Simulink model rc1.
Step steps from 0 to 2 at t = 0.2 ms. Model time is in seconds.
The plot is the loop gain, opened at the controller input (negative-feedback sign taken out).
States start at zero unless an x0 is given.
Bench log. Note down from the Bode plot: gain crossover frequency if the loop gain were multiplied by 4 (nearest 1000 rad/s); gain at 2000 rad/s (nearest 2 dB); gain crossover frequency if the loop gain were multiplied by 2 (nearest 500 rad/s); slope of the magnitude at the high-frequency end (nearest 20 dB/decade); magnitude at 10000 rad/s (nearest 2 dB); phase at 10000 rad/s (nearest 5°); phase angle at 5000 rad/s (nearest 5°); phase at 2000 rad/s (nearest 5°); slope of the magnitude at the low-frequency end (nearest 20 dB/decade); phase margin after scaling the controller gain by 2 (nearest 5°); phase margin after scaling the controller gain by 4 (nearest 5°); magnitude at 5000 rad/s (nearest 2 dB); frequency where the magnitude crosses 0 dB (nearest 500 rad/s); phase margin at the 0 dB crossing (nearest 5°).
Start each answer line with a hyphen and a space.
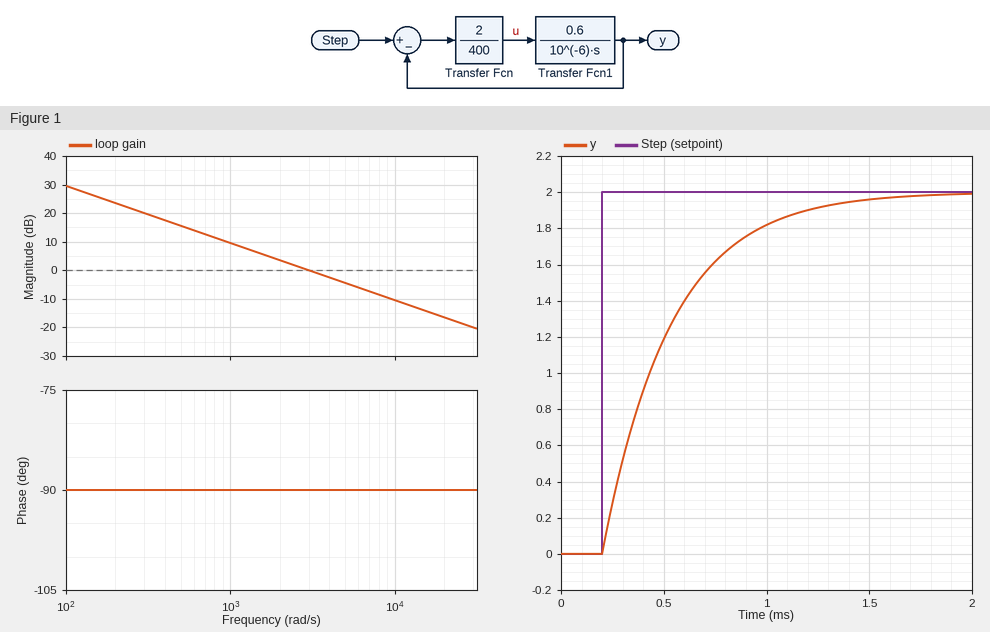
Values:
- 12000 rad/s
- 4 dB
- 6000 rad/s
- -20 dB/decade
- -10 dB
- -90°
- -90°
- -90°
- -20 dB/decade
- 90°
- 90°
- -4 dB
- 3000 rad/s
- 90°
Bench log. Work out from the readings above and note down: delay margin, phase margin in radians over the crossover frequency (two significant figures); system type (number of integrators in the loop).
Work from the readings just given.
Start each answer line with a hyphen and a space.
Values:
- 0.00052 s
- 1
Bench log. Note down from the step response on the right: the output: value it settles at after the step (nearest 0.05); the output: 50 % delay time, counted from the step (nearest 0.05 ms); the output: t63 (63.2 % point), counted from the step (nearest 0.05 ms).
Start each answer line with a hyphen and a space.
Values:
- 2.00
- 0.25 ms
- 0.35 ms
